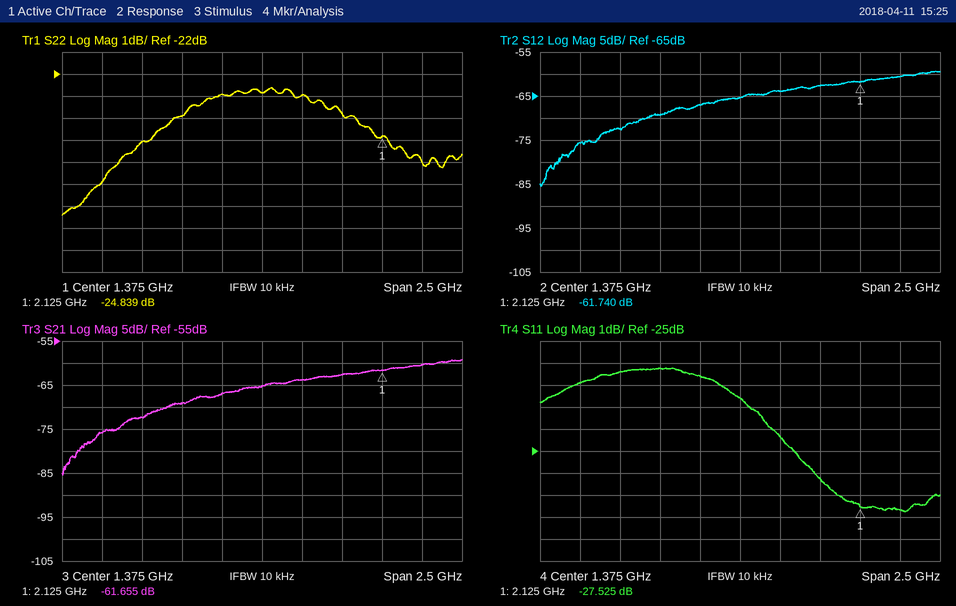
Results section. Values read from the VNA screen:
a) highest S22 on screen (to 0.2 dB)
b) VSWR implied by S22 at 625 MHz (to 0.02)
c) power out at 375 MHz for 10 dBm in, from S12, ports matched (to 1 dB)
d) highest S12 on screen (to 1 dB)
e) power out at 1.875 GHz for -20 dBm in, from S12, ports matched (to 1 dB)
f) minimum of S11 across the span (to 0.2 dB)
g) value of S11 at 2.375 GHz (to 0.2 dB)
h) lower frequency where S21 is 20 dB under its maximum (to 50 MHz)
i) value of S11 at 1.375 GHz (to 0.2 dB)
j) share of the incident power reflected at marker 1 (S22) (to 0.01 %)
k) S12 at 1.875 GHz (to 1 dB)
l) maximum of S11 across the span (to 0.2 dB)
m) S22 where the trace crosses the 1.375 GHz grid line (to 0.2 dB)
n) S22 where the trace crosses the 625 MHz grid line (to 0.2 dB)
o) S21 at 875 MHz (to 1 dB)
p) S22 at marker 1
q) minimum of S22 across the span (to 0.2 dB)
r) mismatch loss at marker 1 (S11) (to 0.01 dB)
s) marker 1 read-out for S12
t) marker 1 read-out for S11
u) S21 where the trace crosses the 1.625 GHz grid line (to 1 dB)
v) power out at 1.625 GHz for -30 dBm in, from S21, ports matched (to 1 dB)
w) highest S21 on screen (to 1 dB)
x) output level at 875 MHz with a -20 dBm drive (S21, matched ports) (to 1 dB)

-22.6 dB
1.12
-66 dBm
-59 dB
-83 dBm
-27.8 dB
-27.6 dB
250 MHz
-22.6 dB
0.33 %
-63 dB
-21.2 dB
-22.8 dB
-25.0 dB
-69 dB
-24.839 dB
-28.4 dB
0.01 dB
-61.740 dB
-27.525 dB
-64 dB
-94 dBm
-59 dB
-89 dBm
